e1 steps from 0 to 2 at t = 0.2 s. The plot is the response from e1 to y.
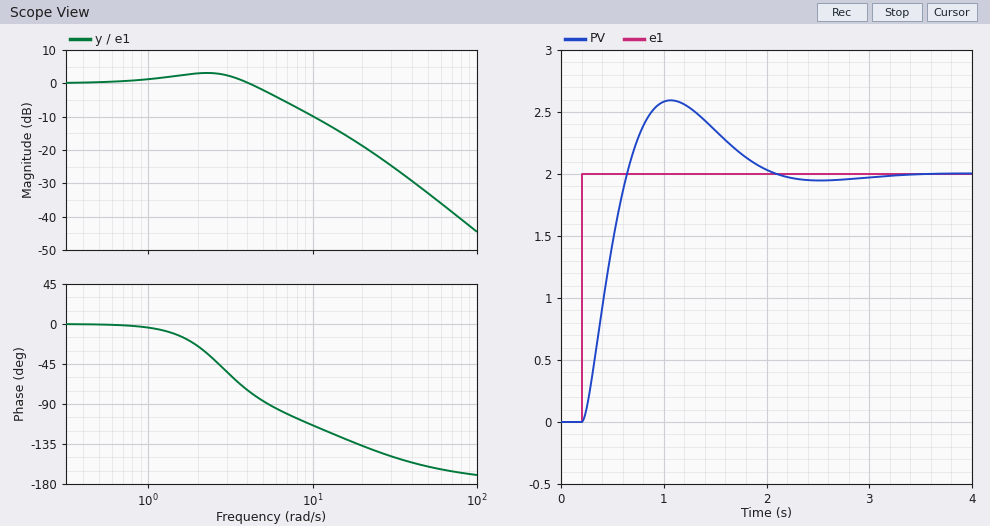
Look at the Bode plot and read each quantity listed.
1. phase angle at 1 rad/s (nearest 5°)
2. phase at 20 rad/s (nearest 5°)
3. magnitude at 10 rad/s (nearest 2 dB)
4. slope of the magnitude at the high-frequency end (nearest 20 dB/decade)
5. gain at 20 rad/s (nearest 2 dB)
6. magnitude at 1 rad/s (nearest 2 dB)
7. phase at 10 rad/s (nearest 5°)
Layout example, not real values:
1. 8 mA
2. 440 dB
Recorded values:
1. -5°
2. -135°
3. -10 dB
4. -40 dB/decade
5. -18 dB
6. 2 dB
7. -115°
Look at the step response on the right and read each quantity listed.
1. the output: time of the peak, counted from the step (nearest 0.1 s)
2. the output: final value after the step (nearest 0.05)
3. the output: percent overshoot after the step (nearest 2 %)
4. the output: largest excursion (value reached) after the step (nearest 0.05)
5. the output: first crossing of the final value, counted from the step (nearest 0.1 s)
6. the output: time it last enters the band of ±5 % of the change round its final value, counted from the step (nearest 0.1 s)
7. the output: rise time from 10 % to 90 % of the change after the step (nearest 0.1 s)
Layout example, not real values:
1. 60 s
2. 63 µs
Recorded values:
1. 0.9 s
2. 2.00
3. 30 %
4. 2.60
5. 0.4 s
6. 1.7 s
7. 0.3 s
